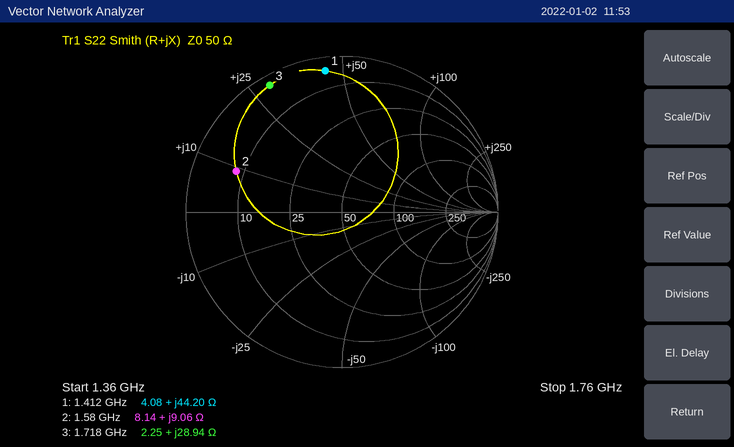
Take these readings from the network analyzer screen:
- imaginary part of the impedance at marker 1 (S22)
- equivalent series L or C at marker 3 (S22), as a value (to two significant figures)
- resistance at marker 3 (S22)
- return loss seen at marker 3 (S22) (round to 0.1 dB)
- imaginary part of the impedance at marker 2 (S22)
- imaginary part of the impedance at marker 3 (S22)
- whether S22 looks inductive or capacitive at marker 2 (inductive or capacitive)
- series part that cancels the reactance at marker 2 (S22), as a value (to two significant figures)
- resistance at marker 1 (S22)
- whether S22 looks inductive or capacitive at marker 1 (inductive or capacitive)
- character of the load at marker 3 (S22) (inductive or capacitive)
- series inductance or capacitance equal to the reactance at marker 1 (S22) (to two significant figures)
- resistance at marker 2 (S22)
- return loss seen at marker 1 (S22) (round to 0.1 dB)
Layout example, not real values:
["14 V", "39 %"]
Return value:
["+44.20 Ω", "2.7 nH", "2.25 Ω", "0.6 dB", "+9.06 Ω", "+28.94 Ω", "inductive", "11 pF", "4.08 Ω", "inductive", "inductive", "5.0 nH", "8.14 Ω", "0.8 dB"]
